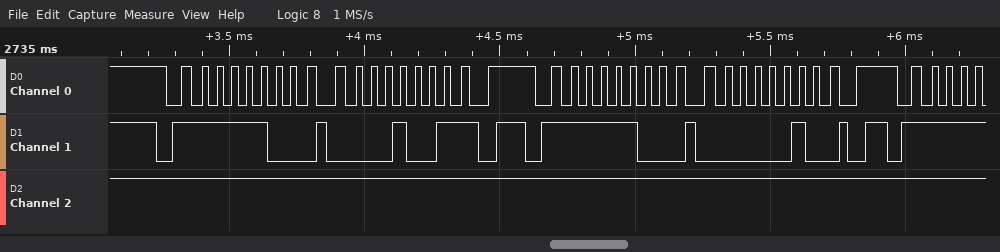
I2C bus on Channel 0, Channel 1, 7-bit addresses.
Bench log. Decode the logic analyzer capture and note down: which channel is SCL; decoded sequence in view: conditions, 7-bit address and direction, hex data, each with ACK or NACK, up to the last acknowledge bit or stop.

Channel 0
start, address 7E write ACK, 09 NACK, stop, start, address 7E write ACK, 02 ACK, stop
